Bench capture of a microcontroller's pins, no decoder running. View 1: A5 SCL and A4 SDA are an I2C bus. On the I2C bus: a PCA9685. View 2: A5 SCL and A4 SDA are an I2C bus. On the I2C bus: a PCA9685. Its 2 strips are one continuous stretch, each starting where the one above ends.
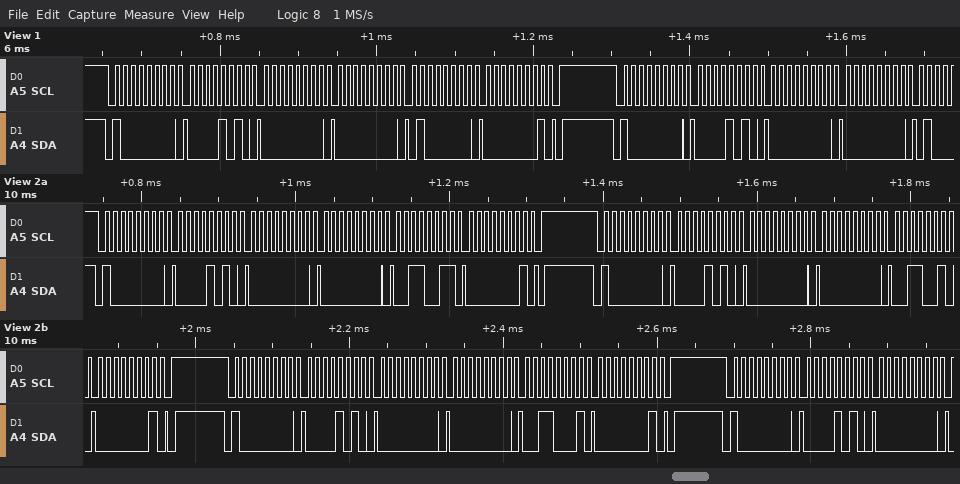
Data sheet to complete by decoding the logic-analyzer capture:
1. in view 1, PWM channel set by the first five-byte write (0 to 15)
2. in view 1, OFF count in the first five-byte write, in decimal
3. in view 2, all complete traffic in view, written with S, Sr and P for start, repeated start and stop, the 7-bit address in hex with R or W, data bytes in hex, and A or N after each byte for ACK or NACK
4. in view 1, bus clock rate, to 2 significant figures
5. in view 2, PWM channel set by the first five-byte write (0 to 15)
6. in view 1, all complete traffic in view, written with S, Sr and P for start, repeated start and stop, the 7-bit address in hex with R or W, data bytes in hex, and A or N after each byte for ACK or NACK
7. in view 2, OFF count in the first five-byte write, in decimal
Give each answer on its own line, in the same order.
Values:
1
320
S 40W A 0A A 00 A 00 A 33 A 01 A P S 40W A 0A A 00 A 00 A 32 A 01 A P S 40W A 0A A 00 A 00 A 31 A 01 A P S 40W A 0A A 00 A
100 kHz
1
S 40W A 0A A 00 A 00 A 40 A 01 A P S 40W A 0A A 00 A 00 A
307
